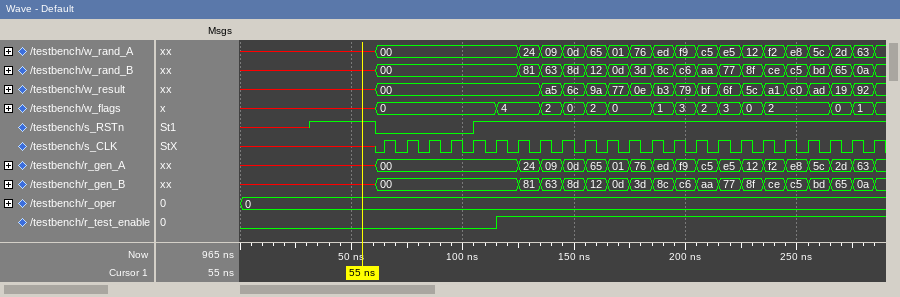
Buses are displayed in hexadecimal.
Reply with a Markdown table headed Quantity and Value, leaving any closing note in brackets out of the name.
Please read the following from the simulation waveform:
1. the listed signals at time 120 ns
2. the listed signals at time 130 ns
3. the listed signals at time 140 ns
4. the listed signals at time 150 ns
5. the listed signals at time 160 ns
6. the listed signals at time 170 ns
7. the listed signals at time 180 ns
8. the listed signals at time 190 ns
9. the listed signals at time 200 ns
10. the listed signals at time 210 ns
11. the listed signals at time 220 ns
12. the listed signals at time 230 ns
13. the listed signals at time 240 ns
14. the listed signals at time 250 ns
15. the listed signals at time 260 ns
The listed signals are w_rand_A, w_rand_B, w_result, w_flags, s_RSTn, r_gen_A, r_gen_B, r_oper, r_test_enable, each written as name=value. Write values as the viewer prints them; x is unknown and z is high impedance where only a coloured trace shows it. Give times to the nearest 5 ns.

| Quantity | Value |
|---|---|
| the listed signals at time 120 ns | w_rand_A=00, w_rand_B=00, w_result=00, w_flags=4, s_RSTn=1, r_gen_A=00, r_gen_B=00, r_oper=0, r_test_enable=1 |
| the listed signals at time 130 ns | w_rand_A=24, w_rand_B=81, w_result=00, w_flags=4, s_RSTn=1, r_gen_A=24, r_gen_B=81, r_oper=0, r_test_enable=1 |
| the listed signals at time 140 ns | w_rand_A=09, w_rand_B=63, w_result=a5, w_flags=2, s_RSTn=1, r_gen_A=09, r_gen_B=63, r_oper=0, r_test_enable=1 |
| the listed signals at time 150 ns | w_rand_A=0d, w_rand_B=8d, w_result=6c, w_flags=0, s_RSTn=1, r_gen_A=0d, r_gen_B=8d, r_oper=0, r_test_enable=1 |
| the listed signals at time 160 ns | w_rand_A=65, w_rand_B=12, w_result=9a, w_flags=2, s_RSTn=1, r_gen_A=65, r_gen_B=12, r_oper=0, r_test_enable=1 |
| the listed signals at time 170 ns | w_rand_A=01, w_rand_B=0d, w_result=77, w_flags=0, s_RSTn=1, r_gen_A=01, r_gen_B=0d, r_oper=0, r_test_enable=1 |
| the listed signals at time 180 ns | w_rand_A=76, w_rand_B=3d, w_result=0e, w_flags=0, s_RSTn=1, r_gen_A=76, r_gen_B=3d, r_oper=0, r_test_enable=1 |
| the listed signals at time 190 ns | w_rand_A=ed, w_rand_B=8c, w_result=b3, w_flags=1, s_RSTn=1, r_gen_A=ed, r_gen_B=8c, r_oper=0, r_test_enable=1 |
| the listed signals at time 200 ns | w_rand_A=f9, w_rand_B=c6, w_result=79, w_flags=3, s_RSTn=1, r_gen_A=f9, r_gen_B=c6, r_oper=0, r_test_enable=1 |
| the listed signals at time 210 ns | w_rand_A=c5, w_rand_B=aa, w_result=bf, w_flags=2, s_RSTn=1, r_gen_A=c5, r_gen_B=aa, r_oper=0, r_test_enable=1 |
| the listed signals at time 220 ns | w_rand_A=e5, w_rand_B=77, w_result=6f, w_flags=3, s_RSTn=1, r_gen_A=e5, r_gen_B=77, r_oper=0, r_test_enable=1 |
| the listed signals at time 230 ns | w_rand_A=12, w_rand_B=8f, w_result=5c, w_flags=0, s_RSTn=1, r_gen_A=12, r_gen_B=8f, r_oper=0, r_test_enable=1 |
| the listed signals at time 240 ns | w_rand_A=f2, w_rand_B=ce, w_result=a1, w_flags=2, s_RSTn=1, r_gen_A=f2, r_gen_B=ce, r_oper=0, r_test_enable=1 |
| the listed signals at time 250 ns | w_rand_A=e8, w_rand_B=c5, w_result=c0, w_flags=2, s_RSTn=1, r_gen_A=e8, r_gen_B=c5, r_oper=0, r_test_enable=1 |
| the listed signals at time 260 ns | w_rand_A=5c, w_rand_B=bd, w_result=ad, w_flags=2, s_RSTn=1, r_gen_A=5c, r_gen_B=bd, r_oper=0, r_test_enable=1 |
